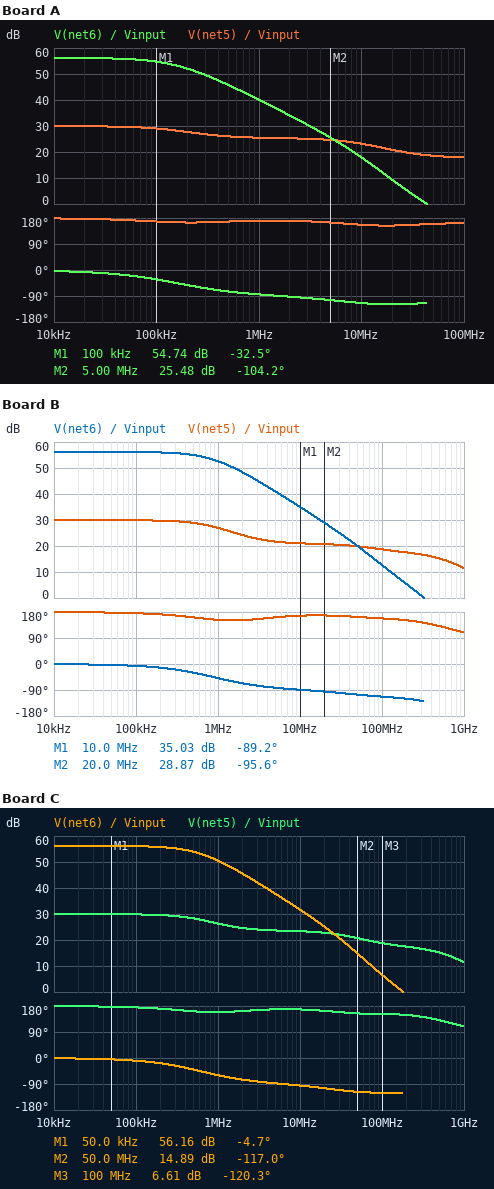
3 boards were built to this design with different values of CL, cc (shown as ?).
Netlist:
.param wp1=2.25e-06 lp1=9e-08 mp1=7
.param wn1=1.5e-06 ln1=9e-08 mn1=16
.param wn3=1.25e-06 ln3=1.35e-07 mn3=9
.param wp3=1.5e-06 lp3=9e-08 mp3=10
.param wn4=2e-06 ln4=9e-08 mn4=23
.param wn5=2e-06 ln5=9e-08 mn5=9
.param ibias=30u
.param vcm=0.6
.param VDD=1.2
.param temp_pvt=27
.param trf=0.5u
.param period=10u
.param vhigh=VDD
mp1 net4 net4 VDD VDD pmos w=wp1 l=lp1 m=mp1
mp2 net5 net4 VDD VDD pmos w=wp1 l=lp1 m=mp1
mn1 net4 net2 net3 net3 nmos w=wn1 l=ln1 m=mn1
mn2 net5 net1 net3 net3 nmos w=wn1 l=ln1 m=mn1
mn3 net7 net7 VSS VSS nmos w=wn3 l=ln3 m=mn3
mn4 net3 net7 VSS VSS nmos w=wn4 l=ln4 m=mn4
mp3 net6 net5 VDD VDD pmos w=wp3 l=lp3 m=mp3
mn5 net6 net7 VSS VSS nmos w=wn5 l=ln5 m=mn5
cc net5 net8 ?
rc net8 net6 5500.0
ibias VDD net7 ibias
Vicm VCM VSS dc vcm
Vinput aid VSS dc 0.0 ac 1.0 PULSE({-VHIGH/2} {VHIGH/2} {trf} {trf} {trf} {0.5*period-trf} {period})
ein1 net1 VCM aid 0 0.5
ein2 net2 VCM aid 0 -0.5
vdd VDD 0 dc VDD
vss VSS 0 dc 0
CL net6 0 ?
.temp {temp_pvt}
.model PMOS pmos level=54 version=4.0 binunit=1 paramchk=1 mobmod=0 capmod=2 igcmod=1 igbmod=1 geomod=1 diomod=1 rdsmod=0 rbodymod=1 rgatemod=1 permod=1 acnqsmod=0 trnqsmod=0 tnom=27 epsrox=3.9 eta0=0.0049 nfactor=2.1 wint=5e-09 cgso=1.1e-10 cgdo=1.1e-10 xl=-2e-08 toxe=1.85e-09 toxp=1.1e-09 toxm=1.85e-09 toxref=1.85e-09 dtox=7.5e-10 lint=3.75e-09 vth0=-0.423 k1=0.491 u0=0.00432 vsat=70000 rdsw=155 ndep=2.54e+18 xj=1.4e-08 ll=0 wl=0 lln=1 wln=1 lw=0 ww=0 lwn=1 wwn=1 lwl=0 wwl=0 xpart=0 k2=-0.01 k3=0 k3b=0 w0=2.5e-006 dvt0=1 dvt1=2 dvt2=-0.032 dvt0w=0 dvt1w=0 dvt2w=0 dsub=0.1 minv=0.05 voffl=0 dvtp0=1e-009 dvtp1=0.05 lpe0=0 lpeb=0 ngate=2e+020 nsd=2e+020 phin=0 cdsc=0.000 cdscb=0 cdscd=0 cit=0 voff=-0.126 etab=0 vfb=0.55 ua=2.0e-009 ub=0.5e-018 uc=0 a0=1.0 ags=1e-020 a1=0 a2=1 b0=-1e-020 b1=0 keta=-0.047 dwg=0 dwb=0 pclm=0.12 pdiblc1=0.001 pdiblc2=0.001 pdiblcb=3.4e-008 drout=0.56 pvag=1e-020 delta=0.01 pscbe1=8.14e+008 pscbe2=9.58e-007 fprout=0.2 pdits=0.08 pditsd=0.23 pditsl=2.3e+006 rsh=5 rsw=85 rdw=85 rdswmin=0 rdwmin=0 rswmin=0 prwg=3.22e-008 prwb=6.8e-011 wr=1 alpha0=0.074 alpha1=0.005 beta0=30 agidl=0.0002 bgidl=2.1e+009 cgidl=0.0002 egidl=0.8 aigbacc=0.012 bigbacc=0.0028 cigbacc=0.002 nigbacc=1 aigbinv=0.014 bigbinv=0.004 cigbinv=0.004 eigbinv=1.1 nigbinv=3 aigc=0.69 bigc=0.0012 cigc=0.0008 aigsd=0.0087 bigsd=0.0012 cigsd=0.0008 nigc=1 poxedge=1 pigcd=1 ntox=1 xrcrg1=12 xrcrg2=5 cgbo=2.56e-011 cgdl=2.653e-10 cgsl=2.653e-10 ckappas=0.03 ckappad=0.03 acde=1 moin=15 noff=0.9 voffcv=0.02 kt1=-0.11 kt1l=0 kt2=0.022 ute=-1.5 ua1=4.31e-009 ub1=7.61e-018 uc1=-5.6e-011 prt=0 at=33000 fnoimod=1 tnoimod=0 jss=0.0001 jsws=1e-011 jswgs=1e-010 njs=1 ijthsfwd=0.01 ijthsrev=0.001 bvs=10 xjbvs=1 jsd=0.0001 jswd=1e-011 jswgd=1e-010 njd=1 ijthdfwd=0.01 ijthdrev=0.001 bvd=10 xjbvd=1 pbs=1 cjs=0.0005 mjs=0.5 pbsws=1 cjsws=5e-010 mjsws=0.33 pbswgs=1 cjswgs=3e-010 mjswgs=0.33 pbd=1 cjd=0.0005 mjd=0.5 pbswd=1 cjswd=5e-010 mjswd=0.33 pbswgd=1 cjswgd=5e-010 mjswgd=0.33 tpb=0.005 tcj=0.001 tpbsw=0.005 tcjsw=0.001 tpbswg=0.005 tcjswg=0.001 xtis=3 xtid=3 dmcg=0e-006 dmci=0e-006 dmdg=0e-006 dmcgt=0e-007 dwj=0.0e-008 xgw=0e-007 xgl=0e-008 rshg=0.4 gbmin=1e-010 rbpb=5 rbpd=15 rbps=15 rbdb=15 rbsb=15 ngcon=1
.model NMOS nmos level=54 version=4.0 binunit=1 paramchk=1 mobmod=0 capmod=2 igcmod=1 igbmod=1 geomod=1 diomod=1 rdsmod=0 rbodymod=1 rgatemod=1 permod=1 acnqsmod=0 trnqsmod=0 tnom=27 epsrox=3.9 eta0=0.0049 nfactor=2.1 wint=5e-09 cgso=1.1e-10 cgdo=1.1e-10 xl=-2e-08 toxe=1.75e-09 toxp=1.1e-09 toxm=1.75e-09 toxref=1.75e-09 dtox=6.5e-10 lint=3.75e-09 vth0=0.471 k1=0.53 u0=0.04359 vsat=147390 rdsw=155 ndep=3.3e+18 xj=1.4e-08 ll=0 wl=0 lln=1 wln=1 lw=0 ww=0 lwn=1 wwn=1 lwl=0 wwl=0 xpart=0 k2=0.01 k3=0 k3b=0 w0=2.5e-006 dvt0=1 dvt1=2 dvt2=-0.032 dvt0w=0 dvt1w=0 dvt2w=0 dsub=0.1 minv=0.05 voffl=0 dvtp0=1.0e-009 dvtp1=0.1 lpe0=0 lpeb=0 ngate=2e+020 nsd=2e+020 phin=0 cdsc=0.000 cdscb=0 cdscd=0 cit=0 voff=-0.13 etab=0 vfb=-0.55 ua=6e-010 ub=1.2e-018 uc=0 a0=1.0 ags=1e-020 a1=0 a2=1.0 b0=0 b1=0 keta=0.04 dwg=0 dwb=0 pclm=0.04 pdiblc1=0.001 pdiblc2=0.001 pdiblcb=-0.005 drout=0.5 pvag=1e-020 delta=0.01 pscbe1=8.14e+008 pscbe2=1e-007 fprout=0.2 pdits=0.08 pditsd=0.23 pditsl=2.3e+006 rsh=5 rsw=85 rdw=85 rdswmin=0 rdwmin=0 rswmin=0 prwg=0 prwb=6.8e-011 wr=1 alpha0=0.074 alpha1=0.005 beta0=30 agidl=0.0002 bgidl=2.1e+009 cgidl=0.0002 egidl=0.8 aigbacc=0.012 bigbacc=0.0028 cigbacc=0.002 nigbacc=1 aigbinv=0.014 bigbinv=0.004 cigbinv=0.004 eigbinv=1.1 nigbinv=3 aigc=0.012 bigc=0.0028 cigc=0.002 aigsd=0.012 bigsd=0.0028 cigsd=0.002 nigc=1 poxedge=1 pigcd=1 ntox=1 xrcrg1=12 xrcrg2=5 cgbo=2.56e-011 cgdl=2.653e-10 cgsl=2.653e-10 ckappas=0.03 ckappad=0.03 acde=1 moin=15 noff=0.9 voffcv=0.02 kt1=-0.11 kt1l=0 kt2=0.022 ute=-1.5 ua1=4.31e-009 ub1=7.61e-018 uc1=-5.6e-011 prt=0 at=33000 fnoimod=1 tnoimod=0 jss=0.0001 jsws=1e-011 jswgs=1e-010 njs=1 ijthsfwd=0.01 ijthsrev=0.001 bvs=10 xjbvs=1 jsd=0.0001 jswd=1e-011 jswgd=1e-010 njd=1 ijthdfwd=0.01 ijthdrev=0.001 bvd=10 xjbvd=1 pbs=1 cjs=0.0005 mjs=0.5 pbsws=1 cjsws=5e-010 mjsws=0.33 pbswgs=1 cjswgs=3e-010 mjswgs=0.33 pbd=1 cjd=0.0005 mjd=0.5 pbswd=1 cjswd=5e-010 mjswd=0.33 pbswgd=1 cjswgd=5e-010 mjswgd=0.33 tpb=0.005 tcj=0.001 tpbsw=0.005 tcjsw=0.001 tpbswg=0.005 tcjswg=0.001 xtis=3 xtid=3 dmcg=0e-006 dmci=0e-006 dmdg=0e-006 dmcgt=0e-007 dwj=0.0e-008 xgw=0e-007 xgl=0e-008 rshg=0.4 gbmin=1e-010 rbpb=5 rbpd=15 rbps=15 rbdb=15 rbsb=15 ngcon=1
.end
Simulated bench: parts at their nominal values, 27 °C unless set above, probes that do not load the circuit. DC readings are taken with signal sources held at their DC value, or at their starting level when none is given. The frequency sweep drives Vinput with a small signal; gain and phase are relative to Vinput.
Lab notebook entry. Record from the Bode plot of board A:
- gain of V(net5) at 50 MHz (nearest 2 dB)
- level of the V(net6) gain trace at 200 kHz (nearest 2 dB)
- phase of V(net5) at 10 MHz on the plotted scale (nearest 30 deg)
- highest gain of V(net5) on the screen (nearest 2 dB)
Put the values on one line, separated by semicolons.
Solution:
18 dB; 52 dB; 150 deg; 30 dB
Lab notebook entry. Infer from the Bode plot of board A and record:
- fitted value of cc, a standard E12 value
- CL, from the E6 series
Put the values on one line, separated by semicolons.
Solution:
1.2 pF; 33 pF
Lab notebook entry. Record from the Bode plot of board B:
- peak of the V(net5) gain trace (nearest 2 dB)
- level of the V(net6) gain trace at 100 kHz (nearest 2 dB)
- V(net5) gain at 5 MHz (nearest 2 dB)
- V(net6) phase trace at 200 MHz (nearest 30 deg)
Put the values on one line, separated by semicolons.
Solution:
30 dB; 56 dB; 22 dB; -120 deg
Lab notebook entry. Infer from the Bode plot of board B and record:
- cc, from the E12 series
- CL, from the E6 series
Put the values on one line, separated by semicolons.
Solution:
330 fF; 3.3 pF
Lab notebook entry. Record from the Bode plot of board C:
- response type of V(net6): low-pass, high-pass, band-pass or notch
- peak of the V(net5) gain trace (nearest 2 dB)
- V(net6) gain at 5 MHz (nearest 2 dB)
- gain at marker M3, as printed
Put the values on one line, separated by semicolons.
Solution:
low-pass; 30 dB; 38 dB; 6.61 dB
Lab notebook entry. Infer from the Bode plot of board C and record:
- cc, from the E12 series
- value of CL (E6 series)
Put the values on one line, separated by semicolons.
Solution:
390 fF; 6.8 pF
